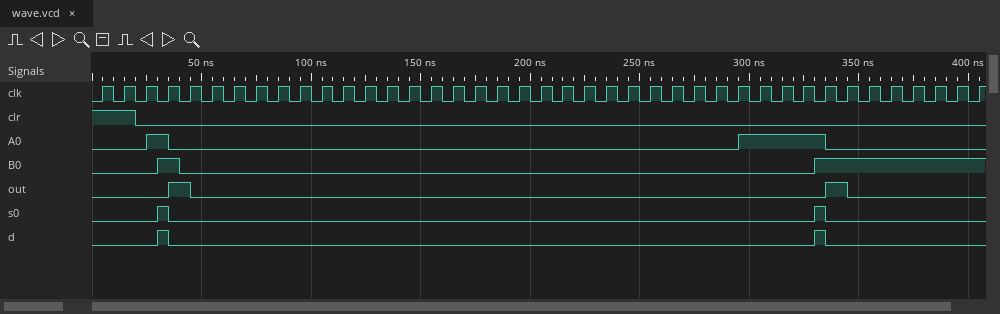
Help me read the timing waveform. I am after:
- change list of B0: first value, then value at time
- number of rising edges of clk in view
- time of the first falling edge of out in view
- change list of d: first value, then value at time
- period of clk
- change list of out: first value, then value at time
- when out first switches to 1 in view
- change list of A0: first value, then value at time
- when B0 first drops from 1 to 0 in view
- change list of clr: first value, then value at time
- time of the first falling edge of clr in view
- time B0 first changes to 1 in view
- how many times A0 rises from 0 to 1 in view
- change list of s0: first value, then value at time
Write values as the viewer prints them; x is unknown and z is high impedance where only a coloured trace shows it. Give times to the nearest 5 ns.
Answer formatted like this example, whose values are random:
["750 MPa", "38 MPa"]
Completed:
["0, 1 at 30 ns, 0 at 40 ns, 1 at 330 ns", "41", "45 ns", "0, 1 at 30 ns, 0 at 35 ns, 1 at 330 ns, 0 at 335 ns", "10 ns", "0, 1 at 35 ns, 0 at 45 ns, 1 at 335 ns, 0 at 345 ns", "35 ns", "0, 1 at 25 ns, 0 at 35 ns, 1 at 295 ns, 0 at 335 ns", "40 ns", "1, 0 at 20 ns", "20 ns", "30 ns", "2", "0, 1 at 30 ns, 0 at 35 ns, 1 at 330 ns, 0 at 335 ns"]
